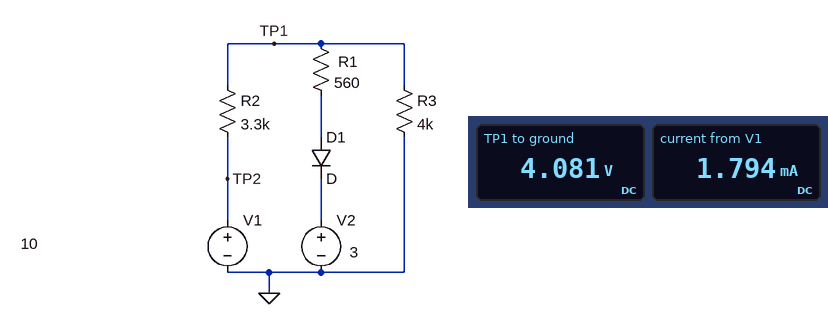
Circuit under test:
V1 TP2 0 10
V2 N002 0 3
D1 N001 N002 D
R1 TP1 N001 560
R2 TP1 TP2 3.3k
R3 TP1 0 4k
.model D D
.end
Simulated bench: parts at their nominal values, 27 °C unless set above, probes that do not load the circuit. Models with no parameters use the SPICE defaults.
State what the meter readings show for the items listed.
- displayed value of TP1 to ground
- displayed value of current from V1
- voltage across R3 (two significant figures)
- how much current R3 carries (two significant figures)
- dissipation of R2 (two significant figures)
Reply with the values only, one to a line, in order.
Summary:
4.081 V
1.794 mA
4.1 V
1.0 mA
11 mW
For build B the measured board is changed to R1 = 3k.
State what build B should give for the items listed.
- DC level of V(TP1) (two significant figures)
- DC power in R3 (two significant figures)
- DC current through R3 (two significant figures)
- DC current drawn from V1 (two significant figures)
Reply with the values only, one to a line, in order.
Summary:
4.8 V
5.7 mW
1.2 mA
1.6 mA
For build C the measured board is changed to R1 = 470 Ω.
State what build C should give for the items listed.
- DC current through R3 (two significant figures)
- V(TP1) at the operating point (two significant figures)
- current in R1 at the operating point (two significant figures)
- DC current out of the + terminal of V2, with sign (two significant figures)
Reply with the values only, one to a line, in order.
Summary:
1.0 mA
4.0 V
800 µA
-800 µA
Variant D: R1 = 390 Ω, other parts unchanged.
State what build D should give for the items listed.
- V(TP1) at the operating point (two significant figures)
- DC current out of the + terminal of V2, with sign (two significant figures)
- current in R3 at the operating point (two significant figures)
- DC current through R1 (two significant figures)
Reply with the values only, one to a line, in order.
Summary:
4.0 V
-830 µA
990 µA
830 µA
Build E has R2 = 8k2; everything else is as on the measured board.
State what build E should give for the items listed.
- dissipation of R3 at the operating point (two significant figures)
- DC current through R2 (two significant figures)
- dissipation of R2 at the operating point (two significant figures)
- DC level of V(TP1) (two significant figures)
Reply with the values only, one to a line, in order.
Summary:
2.7 mW
820 µA
5.5 mW
3.3 V
